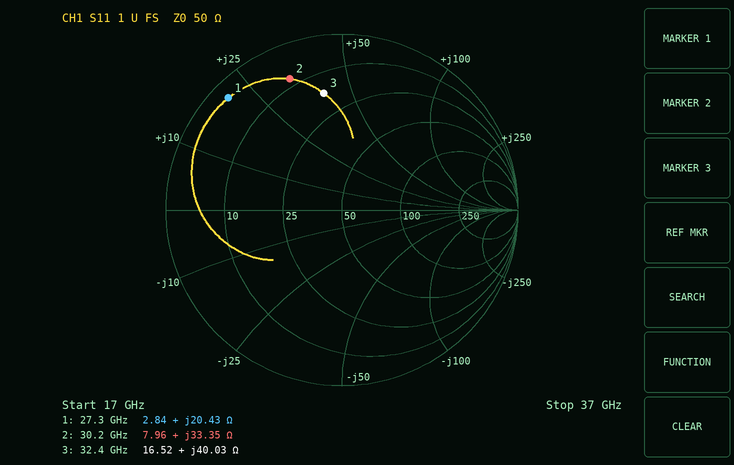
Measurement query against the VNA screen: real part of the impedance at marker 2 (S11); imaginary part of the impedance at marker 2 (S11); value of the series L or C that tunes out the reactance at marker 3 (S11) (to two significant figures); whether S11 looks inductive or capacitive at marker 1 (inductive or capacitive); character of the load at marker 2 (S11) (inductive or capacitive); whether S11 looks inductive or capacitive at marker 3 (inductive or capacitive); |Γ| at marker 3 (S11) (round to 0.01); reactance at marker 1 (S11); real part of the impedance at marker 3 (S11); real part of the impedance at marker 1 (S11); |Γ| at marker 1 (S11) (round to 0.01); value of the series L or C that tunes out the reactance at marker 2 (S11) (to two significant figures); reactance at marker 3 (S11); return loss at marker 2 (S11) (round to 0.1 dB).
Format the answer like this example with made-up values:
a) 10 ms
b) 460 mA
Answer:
a) 7.96 Ω
b) +33.35 Ω
c) 120 fF
d) inductive
e) inductive
f) inductive
g) 0.67
h) +20.43 Ω
i) 16.52 Ω
j) 2.84 Ω
k) 0.91
l) 160 fF
m) +40.03 Ω
n) 1.9 dB
